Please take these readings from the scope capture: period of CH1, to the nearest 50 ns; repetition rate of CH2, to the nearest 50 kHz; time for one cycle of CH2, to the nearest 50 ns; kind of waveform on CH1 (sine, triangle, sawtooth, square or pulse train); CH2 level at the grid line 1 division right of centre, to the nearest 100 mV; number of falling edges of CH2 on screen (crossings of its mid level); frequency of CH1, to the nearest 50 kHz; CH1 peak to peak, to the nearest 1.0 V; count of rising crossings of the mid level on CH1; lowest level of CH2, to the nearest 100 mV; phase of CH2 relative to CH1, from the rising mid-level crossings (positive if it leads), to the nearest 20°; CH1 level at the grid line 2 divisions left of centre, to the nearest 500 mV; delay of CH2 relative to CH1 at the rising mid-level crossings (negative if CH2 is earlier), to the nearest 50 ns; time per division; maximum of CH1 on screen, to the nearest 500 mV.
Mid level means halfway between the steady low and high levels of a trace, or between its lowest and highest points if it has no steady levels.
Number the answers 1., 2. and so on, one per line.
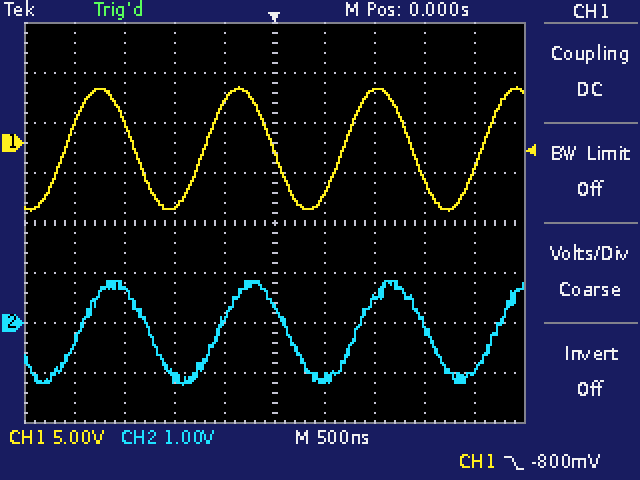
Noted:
1. 1.40 µs
2. 700 kHz
3. 1.40 µs
4. sine
5. -1.1 V
6. 3
7. 700 kHz
8. 12.0 V
9. 4
10. -1.2 V
11. -40°
12. -6.5 V
13. +150 ns
14. 500 ns
15. 5.5 V
